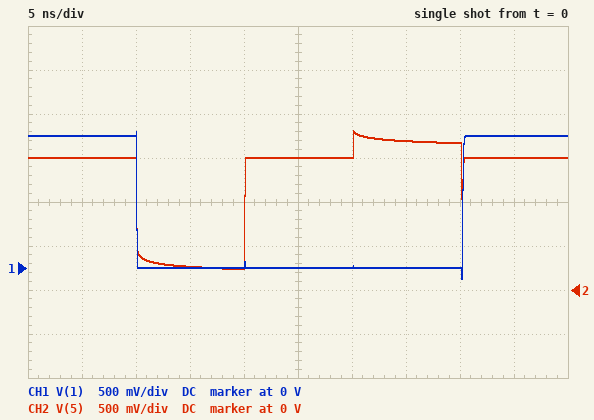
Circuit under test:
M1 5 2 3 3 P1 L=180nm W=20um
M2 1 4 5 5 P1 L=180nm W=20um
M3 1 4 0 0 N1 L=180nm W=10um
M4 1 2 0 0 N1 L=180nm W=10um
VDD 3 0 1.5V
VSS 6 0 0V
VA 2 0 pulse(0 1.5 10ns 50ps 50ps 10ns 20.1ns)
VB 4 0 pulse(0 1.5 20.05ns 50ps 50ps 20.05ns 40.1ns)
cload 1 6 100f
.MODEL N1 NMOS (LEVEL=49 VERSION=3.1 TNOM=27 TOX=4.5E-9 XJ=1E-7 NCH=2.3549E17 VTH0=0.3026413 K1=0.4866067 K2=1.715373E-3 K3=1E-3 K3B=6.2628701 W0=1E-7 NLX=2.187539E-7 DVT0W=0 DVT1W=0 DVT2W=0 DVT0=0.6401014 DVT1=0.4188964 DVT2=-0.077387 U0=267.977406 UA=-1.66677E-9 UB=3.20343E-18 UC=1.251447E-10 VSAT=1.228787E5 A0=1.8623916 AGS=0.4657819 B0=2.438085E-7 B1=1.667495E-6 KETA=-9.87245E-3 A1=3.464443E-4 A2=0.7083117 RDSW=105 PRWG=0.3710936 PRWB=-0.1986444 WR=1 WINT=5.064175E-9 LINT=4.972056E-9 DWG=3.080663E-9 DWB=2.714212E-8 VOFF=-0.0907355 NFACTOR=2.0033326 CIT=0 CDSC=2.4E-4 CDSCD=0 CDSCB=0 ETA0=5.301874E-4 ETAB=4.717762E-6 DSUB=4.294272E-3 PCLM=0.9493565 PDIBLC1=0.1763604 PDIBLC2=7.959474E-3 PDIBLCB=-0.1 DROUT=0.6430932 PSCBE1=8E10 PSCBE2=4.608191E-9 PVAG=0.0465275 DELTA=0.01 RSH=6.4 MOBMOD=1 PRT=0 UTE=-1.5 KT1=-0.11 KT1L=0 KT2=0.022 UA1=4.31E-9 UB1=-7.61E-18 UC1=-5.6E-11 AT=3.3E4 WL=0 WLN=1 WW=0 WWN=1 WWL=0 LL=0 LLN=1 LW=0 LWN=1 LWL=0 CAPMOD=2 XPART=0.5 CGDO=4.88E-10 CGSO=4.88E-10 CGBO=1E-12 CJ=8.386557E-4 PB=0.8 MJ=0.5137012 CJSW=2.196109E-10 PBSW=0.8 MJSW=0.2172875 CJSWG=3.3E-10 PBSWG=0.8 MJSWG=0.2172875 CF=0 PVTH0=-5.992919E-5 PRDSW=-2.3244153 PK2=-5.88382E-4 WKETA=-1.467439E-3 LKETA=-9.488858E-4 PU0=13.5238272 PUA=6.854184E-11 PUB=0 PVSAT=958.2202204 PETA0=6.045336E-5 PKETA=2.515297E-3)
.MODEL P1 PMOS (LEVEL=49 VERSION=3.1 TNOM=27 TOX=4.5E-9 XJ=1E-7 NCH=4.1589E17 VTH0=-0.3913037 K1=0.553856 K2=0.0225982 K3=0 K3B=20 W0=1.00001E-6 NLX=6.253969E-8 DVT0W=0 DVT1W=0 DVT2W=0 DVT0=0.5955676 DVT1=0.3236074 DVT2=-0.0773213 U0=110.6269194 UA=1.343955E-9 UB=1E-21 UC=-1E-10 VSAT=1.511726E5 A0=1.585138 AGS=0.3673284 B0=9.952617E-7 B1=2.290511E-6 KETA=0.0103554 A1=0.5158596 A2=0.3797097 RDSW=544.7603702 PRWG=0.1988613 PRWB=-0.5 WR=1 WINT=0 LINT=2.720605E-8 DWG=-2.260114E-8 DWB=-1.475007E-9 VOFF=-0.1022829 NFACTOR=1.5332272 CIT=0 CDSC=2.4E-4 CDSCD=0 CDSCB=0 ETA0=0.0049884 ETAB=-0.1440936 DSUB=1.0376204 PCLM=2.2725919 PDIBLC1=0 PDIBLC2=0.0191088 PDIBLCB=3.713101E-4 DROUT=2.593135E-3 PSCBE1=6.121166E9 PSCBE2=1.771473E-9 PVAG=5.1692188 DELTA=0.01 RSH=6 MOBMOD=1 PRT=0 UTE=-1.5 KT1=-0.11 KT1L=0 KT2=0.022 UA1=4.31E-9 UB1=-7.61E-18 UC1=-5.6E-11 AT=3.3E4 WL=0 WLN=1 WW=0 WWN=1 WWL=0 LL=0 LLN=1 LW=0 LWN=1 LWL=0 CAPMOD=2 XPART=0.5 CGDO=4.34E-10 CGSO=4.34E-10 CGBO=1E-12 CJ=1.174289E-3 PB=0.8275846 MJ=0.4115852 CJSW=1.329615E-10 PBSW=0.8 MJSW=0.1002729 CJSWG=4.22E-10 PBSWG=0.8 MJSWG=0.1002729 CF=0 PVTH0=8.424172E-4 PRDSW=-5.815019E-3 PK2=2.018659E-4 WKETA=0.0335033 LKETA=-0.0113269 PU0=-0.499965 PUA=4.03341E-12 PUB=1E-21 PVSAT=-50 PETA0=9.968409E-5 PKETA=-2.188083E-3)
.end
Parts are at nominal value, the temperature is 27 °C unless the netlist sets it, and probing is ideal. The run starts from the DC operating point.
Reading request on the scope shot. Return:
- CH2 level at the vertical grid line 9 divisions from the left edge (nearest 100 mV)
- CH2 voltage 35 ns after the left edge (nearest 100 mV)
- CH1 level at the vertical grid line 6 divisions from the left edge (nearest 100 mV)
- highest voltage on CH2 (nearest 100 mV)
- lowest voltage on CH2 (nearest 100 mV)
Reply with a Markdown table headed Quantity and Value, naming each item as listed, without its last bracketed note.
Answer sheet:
| Quantity | Value |
|---|---|
| CH2 level at the vertical grid line 9 divisions from the left edge | 1.5 V |
| CH2 voltage 35 ns after the left edge | 1.7 V |
| CH1 level at the vertical grid line 6 divisions from the left edge | 0 V |
| highest voltage on CH2 | 1.8 V |
| lowest voltage on CH2 | 200 mV |
